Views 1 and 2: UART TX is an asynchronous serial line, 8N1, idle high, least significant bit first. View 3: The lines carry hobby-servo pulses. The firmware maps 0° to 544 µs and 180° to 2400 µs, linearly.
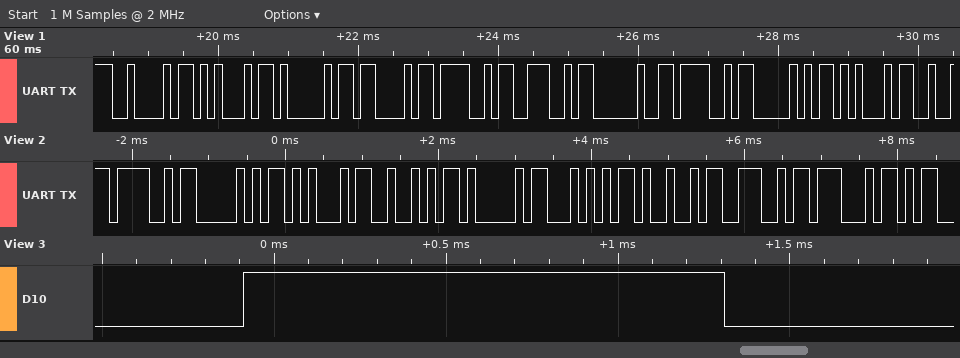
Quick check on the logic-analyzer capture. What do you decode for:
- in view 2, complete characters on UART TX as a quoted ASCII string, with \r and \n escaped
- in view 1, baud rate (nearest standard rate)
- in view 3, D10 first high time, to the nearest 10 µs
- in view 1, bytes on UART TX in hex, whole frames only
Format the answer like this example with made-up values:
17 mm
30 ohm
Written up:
"OPERATING"
9600 baud
1400 µs
0x42 0x45 0x41 0x43 0x4F 0x4E 0x20 0x4F 0x50 0x45
